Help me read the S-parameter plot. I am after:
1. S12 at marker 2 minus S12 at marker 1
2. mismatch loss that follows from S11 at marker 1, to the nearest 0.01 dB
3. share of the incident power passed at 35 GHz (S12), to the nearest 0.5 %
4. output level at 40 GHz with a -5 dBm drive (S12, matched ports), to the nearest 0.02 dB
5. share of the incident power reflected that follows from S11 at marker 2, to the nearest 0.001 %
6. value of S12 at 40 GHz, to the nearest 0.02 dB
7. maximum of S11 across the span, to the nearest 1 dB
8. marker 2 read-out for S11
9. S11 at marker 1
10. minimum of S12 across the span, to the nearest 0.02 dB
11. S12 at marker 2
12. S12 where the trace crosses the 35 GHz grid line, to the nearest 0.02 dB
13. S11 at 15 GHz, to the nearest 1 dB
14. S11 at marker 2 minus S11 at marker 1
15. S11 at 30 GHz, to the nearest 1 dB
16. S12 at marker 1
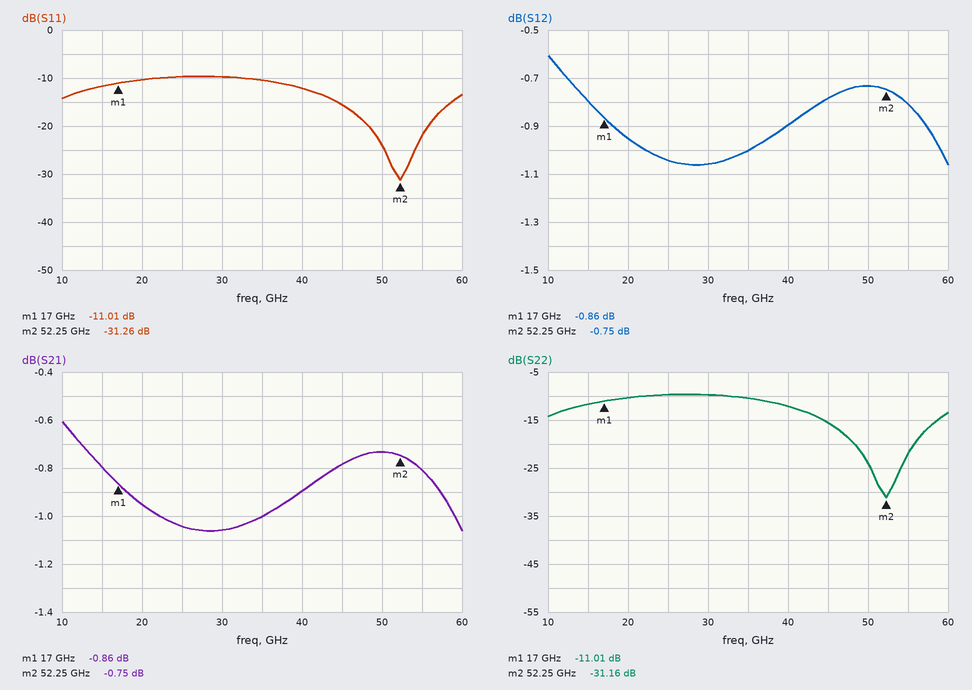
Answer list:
0.11 dB
0.36 dB
79.5 %
-5.90 dBm
0.075 %
-0.90 dB
-10 dB
-31.26 dB
-11.01 dB
-1.06 dB
-0.75 dB
-1.00 dB
-12 dB
-20.25 dB
-10 dB
-0.86 dB
